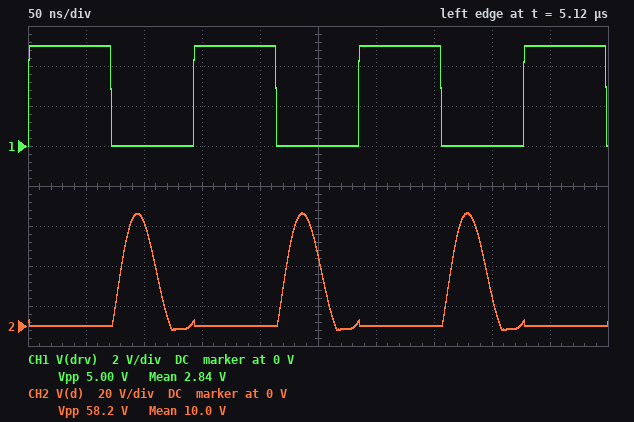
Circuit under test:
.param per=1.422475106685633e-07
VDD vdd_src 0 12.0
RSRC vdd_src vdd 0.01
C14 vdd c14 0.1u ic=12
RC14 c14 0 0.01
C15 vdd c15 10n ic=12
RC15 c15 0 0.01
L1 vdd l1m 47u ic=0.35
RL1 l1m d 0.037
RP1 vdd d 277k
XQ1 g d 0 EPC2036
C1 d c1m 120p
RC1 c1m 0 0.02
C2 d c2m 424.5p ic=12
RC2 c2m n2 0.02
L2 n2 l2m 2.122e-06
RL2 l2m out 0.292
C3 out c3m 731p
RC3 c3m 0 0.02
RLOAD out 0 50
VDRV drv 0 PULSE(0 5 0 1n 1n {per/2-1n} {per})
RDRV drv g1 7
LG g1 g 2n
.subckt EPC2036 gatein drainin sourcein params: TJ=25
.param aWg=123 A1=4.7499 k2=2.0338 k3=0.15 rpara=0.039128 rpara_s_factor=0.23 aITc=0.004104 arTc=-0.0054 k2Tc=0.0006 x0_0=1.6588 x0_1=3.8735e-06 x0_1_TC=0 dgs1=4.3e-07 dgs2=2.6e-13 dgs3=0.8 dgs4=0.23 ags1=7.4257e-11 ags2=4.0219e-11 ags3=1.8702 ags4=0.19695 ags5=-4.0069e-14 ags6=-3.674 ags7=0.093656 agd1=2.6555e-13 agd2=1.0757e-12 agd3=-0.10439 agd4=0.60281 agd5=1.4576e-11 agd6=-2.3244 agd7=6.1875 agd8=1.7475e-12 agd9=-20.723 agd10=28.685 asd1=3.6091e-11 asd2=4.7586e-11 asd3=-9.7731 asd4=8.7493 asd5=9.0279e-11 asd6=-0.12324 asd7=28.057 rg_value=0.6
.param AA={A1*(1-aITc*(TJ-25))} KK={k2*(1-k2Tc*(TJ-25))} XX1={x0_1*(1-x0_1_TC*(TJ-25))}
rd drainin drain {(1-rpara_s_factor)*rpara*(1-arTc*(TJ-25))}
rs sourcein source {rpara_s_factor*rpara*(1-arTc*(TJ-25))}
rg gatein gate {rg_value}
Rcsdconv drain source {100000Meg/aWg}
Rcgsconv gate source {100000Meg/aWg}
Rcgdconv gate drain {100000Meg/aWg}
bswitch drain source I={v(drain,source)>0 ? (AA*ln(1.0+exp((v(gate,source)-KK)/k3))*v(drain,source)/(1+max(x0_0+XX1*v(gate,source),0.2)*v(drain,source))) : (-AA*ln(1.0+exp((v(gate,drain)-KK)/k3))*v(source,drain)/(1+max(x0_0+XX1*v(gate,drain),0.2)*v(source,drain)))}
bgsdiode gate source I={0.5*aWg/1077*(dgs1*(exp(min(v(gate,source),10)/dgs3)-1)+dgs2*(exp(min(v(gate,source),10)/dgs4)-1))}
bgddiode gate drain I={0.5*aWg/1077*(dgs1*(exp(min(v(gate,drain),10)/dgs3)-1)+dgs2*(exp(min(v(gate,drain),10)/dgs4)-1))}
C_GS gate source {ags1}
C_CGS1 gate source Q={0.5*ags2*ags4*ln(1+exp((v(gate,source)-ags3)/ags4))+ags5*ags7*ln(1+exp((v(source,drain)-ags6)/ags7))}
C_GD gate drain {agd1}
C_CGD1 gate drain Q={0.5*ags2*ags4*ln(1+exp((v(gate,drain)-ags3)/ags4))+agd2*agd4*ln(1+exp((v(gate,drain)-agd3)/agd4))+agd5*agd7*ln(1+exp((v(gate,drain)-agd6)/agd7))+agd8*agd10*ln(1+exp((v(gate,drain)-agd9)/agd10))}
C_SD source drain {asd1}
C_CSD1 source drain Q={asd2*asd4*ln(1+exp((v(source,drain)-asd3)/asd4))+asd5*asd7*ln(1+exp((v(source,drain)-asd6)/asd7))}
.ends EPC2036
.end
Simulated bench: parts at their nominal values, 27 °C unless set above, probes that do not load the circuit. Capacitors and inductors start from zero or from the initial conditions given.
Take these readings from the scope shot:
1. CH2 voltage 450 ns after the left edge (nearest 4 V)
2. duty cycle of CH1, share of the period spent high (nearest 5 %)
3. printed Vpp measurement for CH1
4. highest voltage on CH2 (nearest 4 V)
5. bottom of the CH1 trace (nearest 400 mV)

0 V
50 %
5.00 V
56 V
0 V
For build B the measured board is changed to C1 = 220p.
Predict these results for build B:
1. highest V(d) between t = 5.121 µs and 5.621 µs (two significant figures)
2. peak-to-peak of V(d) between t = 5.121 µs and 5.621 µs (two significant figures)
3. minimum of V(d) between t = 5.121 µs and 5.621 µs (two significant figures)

46 V
47 V
-1.4 V
